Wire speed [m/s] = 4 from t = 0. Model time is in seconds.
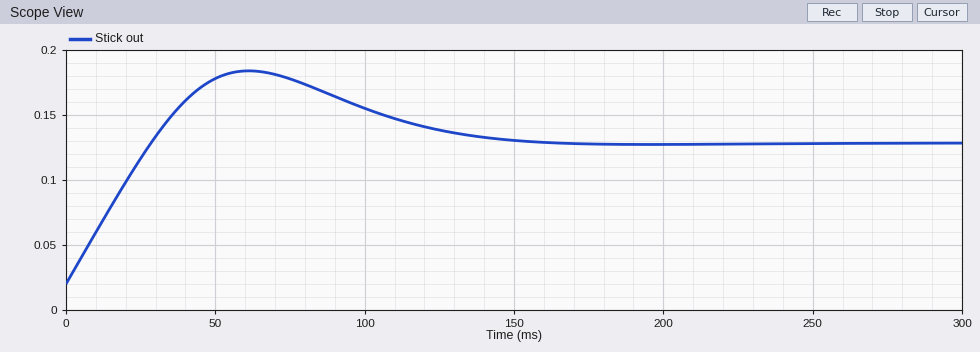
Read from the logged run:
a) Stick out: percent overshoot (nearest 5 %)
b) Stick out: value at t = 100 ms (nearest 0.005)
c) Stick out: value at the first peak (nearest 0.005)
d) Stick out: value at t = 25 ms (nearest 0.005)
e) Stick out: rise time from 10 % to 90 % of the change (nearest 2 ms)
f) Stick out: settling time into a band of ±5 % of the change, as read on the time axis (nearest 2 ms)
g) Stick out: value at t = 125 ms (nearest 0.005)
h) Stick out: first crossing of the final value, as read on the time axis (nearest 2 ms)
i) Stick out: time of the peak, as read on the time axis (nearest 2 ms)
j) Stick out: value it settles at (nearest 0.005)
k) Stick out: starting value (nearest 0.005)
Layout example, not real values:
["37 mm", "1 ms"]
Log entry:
["50 %", "0.155", "0.185", "0.115", "22 ms", "136 ms", "0.140", "28 ms", "62 ms", "0.130", "0.020"]
